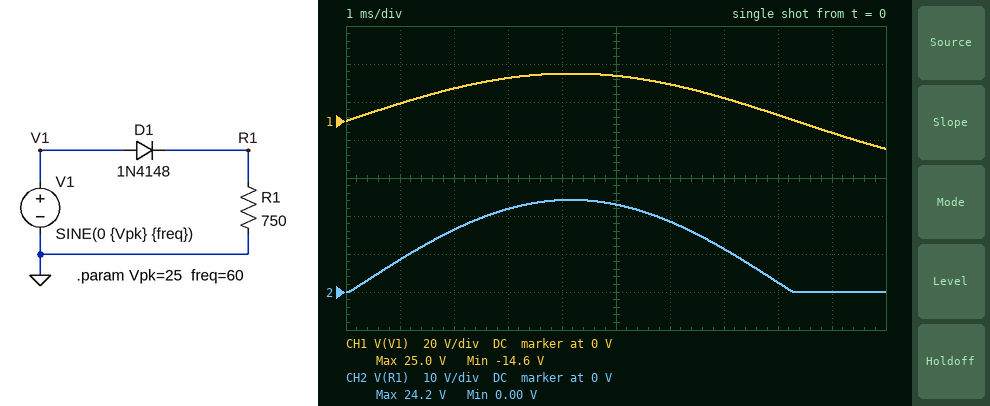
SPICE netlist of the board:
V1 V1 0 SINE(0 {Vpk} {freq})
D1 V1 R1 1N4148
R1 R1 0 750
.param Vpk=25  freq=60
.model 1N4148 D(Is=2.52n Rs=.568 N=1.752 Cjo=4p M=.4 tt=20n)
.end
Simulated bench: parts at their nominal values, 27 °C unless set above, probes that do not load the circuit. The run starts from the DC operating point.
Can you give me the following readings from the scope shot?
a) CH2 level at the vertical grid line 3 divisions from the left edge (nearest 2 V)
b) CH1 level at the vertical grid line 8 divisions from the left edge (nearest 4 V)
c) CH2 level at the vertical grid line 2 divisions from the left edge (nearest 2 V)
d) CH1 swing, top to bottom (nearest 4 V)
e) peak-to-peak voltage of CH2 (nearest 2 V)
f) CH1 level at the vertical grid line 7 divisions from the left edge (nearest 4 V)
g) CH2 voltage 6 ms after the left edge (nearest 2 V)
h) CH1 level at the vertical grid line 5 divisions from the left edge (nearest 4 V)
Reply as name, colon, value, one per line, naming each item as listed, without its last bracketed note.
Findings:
CH2 level at the vertical grid line 3 divisions from the left edge: 22 V
CH1 level at the vertical grid line 8 divisions from the left edge: 4 V
CH2 level at the vertical grid line 2 divisions from the left edge: 16 V
CH1 swing, top to bottom: 40 V
peak-to-peak voltage of CH2: 24 V
CH1 level at the vertical grid line 7 divisions from the left edge: 12 V
CH2 voltage 6 ms after the left edge: 18 V
CH1 level at the vertical grid line 5 divisions from the left edge: 24 V
